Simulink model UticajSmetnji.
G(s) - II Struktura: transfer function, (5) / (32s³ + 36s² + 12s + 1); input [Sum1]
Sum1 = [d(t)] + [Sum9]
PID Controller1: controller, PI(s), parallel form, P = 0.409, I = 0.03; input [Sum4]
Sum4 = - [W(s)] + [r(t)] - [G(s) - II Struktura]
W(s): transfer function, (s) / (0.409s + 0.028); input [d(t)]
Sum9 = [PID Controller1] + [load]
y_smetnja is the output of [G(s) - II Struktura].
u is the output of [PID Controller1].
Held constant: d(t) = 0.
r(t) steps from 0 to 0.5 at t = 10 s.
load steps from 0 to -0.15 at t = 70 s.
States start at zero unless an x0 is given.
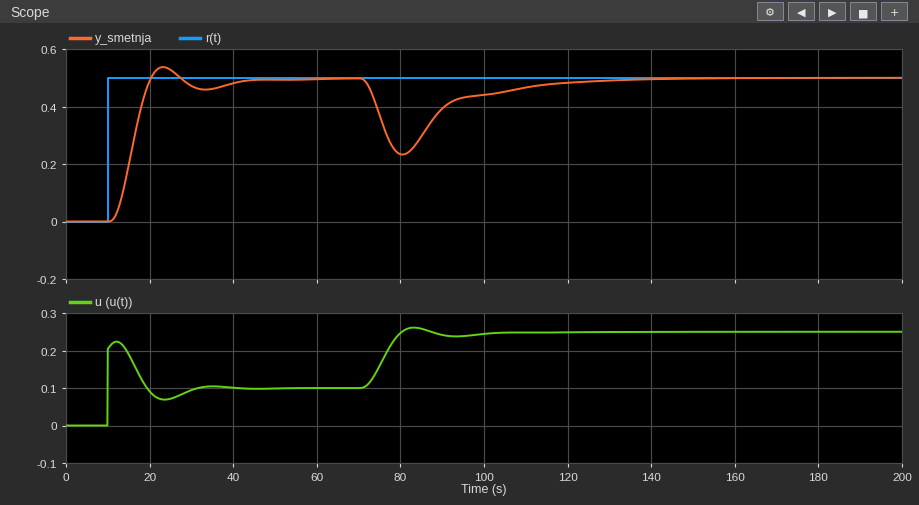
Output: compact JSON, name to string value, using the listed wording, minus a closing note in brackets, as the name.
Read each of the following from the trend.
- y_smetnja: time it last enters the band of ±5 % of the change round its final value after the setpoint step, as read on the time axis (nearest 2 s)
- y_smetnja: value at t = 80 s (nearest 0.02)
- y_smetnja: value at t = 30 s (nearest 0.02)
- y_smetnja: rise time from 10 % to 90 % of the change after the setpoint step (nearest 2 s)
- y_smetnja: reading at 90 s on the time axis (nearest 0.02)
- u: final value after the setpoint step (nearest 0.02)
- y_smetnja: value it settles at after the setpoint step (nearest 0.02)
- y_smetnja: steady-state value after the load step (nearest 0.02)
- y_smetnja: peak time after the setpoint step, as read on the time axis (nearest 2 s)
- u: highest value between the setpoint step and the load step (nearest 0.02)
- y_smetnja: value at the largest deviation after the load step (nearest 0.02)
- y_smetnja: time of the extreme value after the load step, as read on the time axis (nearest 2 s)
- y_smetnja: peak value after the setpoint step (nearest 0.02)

{"y_smetnja: time it last enters the band of ±5 % of the change round its final value after the setpoint step, as read on the time axis": "38 s", "y_smetnja: value at t = 80 s": "0.24", "y_smetnja: value at t = 30 s": "0.48", "y_smetnja: rise time from 10 % to 90 % of the change after the setpoint step": "6 s", "y_smetnja: reading at 90 s on the time axis": "0.40", "u: final value after the setpoint step": "0.10", "y_smetnja: value it settles at after the setpoint step": "0.50", "y_smetnja: steady-state value after the load step": "0.50", "y_smetnja: peak time after the setpoint step, as read on the time axis": "24 s", "u: highest value between the setpoint step and the load step": "0.22", "y_smetnja: value at the largest deviation after the load step": "0.24", "y_smetnja: time of the extreme value after the load step, as read on the time axis": "80 s", "y_smetnja: peak value after the setpoint step": "0.54"}
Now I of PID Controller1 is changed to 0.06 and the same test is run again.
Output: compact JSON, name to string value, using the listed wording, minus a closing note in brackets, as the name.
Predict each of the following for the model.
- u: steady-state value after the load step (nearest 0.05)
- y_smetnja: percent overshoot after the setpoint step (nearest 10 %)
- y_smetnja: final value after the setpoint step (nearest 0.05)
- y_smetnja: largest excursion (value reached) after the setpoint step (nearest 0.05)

{"u: steady-state value after the load step": "0.25", "y_smetnja: percent overshoot after the setpoint step": "30 %", "y_smetnja: final value after the setpoint step": "0.50", "y_smetnja: largest excursion (value reached) after the setpoint step": "0.65"}
